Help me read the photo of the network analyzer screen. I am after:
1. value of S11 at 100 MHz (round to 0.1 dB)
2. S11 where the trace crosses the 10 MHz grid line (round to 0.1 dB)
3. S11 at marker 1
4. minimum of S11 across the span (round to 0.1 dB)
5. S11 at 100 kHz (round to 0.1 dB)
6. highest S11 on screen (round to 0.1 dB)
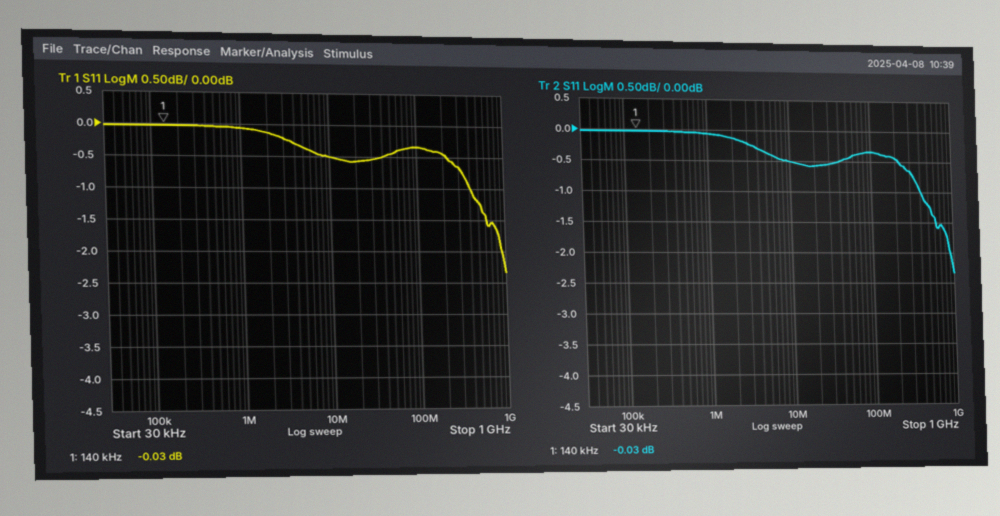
-0.3 dB
-0.5 dB
-0.03 dB
-2.3 dB
0.0 dB
0.0 dB
